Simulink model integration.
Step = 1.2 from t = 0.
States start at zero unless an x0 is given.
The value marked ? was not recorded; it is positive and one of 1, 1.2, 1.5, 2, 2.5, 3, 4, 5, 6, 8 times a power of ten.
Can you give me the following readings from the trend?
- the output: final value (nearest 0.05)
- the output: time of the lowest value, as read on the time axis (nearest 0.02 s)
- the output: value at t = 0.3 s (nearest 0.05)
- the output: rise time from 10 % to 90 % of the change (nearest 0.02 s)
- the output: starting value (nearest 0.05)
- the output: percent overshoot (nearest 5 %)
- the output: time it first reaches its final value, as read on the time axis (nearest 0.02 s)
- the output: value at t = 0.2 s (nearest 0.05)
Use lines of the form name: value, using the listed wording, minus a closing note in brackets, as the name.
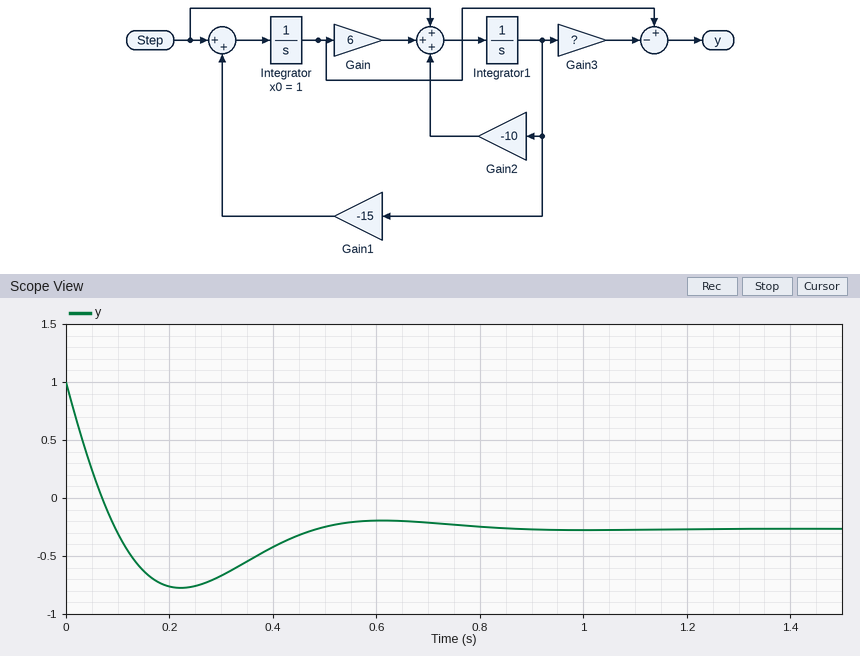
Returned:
the output: final value: -0.25
the output: time of the lowest value, as read on the time axis: 0.22 s
the output: value at t = 0.3 s: -0.65
the output: rise time from 10 % to 90 % of the change: 0.08 s
the output: starting value: 1.00
the output: percent overshoot: 40 %
the output: time it first reaches its final value, as read on the time axis: 0.10 s
the output: value at t = 0.2 s: -0.75
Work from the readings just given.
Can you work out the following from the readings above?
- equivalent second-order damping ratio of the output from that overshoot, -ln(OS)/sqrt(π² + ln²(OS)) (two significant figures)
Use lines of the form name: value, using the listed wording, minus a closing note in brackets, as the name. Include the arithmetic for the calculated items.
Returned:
equivalent second-order damping ratio of the output from that overshoot, -ln(OS)/sqrt(π² + ln²(OS)): ln(0.4) = -0.916; 0.916 / sqrt(9.870 + 0.840) = 0.28
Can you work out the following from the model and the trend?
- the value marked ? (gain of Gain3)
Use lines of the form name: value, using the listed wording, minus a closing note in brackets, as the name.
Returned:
the value marked ?: 2.5
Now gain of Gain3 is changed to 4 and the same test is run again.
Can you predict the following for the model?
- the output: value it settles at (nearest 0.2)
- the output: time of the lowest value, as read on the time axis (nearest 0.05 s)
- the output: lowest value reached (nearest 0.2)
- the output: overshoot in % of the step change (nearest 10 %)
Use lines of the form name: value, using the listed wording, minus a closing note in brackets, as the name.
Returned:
the output: value it settles at: -0.4
the output: time of the lowest value, as read on the time axis: 0.20 s
the output: lowest value reached: -1.4
the output: overshoot in % of the step change: 70 %
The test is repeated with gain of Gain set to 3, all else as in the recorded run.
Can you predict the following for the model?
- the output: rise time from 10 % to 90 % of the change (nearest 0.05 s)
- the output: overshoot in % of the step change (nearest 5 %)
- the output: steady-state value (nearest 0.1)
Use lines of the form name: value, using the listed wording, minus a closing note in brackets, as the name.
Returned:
the output: rise time from 10 % to 90 % of the change: 0.20 s
the output: overshoot in % of the step change: 10 %
the output: steady-state value: -0.3
